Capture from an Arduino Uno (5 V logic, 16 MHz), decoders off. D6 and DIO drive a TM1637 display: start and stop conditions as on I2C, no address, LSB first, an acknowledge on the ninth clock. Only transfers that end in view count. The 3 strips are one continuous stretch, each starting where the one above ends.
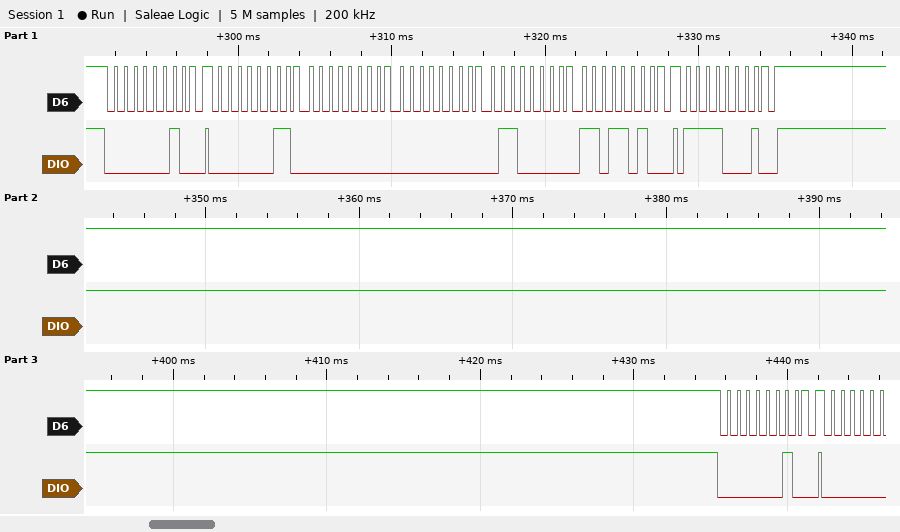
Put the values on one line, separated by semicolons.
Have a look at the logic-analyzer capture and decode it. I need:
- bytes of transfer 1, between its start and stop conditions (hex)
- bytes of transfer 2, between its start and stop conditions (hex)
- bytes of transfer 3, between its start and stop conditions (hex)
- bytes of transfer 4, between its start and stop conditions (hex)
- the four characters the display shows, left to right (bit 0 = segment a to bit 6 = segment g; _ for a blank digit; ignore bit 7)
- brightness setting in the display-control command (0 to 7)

40; C0 00 00 06 5B; 8F; 40; __12; 7
